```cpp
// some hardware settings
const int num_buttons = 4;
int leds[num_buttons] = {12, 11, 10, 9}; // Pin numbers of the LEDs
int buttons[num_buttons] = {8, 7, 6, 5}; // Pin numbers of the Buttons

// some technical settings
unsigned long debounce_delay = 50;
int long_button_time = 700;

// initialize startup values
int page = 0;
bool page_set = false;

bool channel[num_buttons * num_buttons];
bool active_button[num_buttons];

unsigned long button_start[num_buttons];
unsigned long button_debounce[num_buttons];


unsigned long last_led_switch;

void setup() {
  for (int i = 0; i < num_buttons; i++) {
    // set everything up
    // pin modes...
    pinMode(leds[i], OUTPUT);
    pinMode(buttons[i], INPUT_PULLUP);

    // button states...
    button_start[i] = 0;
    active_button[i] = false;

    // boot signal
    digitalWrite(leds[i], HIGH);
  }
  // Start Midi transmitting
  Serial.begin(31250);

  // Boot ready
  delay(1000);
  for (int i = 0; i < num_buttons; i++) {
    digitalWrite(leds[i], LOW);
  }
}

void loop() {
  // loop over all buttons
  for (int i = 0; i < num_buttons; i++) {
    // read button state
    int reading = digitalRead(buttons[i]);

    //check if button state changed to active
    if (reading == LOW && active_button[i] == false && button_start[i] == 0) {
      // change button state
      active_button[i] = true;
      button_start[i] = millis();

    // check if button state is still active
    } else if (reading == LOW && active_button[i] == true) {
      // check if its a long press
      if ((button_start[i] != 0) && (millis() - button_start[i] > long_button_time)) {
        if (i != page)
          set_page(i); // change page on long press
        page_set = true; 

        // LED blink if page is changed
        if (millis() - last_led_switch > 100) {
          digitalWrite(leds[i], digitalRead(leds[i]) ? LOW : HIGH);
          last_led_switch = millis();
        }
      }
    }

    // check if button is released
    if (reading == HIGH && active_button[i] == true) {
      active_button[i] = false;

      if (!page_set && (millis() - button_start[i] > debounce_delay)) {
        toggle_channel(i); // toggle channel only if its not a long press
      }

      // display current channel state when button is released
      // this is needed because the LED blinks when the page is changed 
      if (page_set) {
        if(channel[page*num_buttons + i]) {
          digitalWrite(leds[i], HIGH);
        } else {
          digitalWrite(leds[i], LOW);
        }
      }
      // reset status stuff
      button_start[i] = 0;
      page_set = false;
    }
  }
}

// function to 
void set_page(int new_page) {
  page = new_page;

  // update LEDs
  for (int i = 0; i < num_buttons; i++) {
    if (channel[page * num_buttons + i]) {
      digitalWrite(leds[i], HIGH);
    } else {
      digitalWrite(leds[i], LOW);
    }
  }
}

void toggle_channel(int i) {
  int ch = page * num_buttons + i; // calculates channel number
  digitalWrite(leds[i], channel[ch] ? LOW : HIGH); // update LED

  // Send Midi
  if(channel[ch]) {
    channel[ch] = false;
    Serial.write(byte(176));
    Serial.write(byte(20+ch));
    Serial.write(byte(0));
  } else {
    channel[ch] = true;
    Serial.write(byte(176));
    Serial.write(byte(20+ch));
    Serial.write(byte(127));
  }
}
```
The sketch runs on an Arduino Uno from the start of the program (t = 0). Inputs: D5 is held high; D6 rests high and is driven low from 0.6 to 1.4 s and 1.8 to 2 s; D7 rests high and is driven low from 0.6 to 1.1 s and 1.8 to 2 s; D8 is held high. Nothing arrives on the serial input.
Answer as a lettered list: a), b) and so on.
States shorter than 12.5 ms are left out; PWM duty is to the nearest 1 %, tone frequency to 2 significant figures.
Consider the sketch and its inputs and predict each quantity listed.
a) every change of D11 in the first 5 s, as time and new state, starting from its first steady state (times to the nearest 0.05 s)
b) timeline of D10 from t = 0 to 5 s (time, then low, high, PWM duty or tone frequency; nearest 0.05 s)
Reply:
a) 0 s high; 1 s low; 1.1 s high; 2 s low
b) 0 s high; 1 s low; 1.4 s high; 2 s low
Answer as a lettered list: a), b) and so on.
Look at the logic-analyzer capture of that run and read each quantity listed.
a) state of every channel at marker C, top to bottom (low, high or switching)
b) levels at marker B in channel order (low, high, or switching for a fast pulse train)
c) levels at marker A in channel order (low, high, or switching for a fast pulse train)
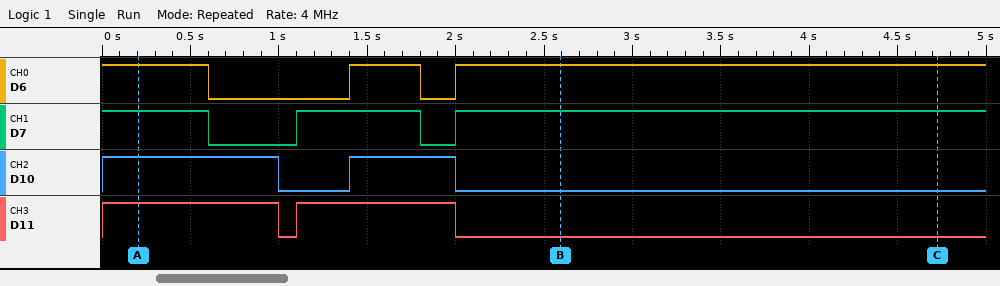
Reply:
a) D6 high, D7 high, D10 low, D11 low
b) D6 high, D7 high, D10 low, D11 low
c) D6 high, D7 high, D10 high, D11 high
